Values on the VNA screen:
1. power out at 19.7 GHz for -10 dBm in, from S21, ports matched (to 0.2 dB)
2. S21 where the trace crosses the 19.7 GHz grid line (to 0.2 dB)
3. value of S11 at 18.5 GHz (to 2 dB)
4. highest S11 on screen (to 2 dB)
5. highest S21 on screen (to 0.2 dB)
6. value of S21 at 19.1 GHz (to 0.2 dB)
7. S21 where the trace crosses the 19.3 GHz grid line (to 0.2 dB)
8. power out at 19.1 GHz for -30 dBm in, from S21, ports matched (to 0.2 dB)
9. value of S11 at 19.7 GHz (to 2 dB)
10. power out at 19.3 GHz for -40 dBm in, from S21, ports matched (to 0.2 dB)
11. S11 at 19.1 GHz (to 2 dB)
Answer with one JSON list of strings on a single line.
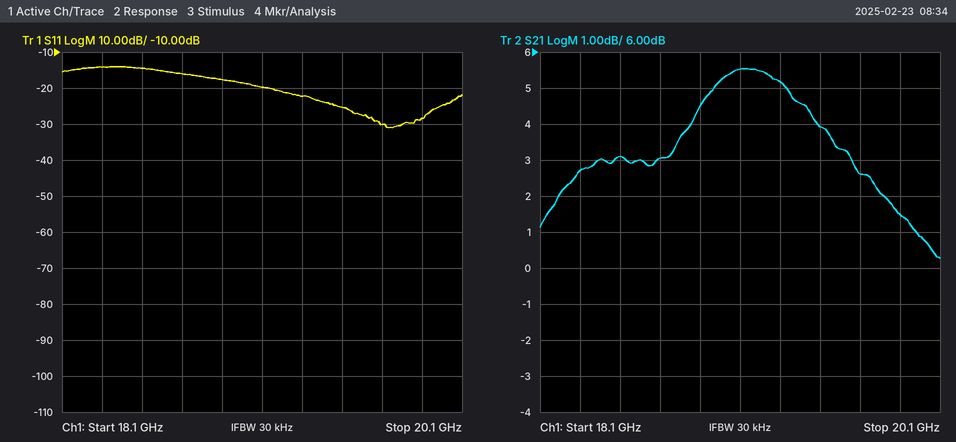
["-7.4 dBm", "2.6 dB", "-14 dB", "-14 dB", "5.6 dB", "5.6 dB", "5.2 dB", "-24.4 dBm", "-30 dB", "-34.8 dBm", "-20 dB"]
